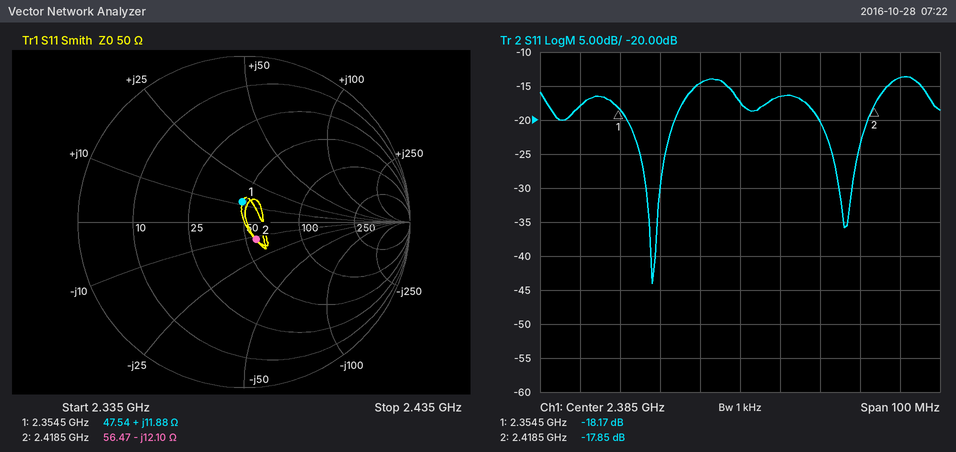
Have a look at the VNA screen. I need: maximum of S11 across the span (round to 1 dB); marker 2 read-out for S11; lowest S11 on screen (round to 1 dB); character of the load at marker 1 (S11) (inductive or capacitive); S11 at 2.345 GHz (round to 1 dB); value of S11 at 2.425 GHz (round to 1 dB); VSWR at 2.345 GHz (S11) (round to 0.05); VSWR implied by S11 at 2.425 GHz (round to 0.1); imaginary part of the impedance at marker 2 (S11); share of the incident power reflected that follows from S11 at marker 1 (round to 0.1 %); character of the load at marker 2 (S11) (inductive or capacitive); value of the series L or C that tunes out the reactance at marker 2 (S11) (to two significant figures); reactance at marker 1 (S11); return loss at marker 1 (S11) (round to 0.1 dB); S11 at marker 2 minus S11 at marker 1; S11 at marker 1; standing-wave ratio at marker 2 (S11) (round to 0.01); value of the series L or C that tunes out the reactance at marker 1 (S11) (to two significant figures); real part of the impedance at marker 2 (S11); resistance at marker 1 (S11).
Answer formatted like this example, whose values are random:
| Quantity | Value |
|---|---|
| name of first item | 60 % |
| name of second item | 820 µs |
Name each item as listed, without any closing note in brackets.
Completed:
| Quantity | Value |
|---|---|
| maximum of S11 across the span | -14 dB |
| marker 2 read-out for S11 | -17.85 dB |
| lowest S11 on screen | -44 dB |
| character of the load at marker 1 (S11) | inductive |
| S11 at 2.345 GHz | -18 dB |
| value of S11 at 2.425 GHz | -14 dB |
| VSWR at 2.345 GHz (S11) | 1.30 |
| VSWR implied by S11 at 2.425 GHz | 1.5 |
| imaginary part of the impedance at marker 2 | -12.10 Ω |
| share of the incident power reflected that follows from S11 at marker 1 | 1.5 % |
| character of the load at marker 2 (S11) | capacitive |
| value of the series L or C that tunes out the reactance at marker 2 (S11) | 800 pH |
| reactance at marker 1 | +11.88 Ω |
| return loss at marker 1 (S11) | 18.2 dB |
| S11 at marker 2 minus S11 at marker 1 | 0.32 dB |
| S11 at marker 1 | -18.17 dB |
| standing-wave ratio at marker 2 (S11) | 1.29 |
| value of the series L or C that tunes out the reactance at marker 1 (S11) | 5.7 pF |
| real part of the impedance at marker 2 | 56.47 Ω |
| resistance at marker 1 | 47.54 Ω |
